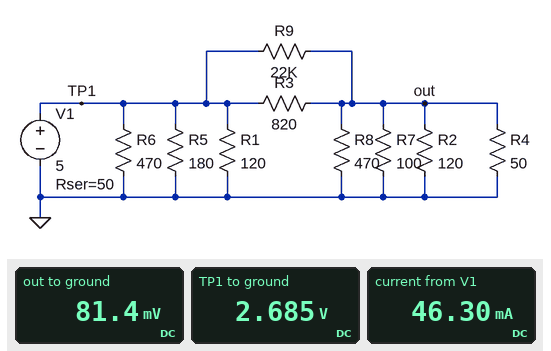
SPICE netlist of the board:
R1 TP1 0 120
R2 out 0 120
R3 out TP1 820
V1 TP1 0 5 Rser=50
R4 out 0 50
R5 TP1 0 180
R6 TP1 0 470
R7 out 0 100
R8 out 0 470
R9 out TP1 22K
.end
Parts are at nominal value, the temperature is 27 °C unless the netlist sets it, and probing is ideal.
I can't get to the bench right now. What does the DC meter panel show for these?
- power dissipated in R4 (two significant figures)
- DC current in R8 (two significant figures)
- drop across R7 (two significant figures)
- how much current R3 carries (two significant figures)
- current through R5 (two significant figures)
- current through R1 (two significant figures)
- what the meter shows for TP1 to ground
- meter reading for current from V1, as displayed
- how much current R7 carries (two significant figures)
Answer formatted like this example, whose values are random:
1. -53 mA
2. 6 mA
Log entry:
1. 130 µW
2. 170 µA
3. 81 mV
4. 3.2 mA
5. 15 mA
6. 22 mA
7. 2.685 V
8. 46.30 mA
9. 810 µA
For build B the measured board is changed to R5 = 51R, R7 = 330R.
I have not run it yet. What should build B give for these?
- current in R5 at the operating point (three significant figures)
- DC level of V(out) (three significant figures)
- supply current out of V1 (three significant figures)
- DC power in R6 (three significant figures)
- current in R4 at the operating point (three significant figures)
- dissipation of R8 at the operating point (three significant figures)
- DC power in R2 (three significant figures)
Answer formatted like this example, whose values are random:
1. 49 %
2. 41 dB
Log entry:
1. 38.2 mA
2. 71.0 mV
3. 61.0 mA
4. 8.09 mW
5. 1.42 mA
6. 10.7 µW
7. 42.0 µW
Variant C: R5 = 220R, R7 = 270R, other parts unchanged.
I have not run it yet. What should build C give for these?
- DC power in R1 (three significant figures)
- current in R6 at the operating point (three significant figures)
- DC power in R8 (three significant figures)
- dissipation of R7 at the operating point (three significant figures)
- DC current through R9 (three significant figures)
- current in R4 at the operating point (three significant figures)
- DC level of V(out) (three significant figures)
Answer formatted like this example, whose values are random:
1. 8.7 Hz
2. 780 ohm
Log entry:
1. 63.5 mW
2. 5.87 mA
3. 20.7 µW
4. 36.0 µW
5. 121 µA
6. 1.97 mA
7. 98.6 mV
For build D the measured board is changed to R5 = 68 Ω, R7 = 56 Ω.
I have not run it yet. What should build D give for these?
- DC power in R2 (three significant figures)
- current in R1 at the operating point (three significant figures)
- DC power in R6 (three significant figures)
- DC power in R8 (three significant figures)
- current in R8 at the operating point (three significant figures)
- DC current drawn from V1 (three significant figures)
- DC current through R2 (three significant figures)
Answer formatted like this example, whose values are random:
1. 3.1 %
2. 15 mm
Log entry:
1. 25.2 µW
2. 18.0 mA
3. 9.88 mW
4. 6.43 µW
5. 117 µA
6. 56.9 mA
7. 458 µA
